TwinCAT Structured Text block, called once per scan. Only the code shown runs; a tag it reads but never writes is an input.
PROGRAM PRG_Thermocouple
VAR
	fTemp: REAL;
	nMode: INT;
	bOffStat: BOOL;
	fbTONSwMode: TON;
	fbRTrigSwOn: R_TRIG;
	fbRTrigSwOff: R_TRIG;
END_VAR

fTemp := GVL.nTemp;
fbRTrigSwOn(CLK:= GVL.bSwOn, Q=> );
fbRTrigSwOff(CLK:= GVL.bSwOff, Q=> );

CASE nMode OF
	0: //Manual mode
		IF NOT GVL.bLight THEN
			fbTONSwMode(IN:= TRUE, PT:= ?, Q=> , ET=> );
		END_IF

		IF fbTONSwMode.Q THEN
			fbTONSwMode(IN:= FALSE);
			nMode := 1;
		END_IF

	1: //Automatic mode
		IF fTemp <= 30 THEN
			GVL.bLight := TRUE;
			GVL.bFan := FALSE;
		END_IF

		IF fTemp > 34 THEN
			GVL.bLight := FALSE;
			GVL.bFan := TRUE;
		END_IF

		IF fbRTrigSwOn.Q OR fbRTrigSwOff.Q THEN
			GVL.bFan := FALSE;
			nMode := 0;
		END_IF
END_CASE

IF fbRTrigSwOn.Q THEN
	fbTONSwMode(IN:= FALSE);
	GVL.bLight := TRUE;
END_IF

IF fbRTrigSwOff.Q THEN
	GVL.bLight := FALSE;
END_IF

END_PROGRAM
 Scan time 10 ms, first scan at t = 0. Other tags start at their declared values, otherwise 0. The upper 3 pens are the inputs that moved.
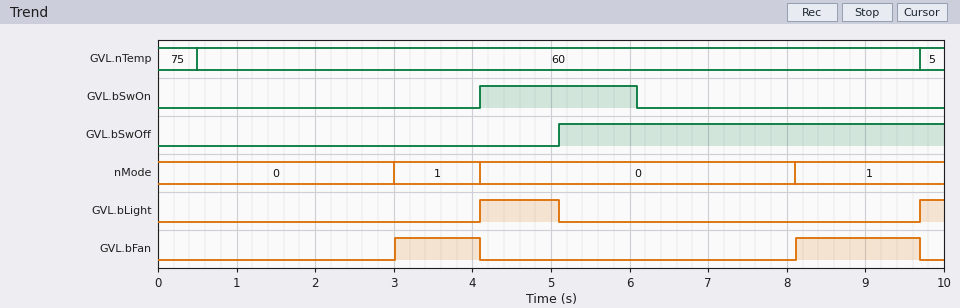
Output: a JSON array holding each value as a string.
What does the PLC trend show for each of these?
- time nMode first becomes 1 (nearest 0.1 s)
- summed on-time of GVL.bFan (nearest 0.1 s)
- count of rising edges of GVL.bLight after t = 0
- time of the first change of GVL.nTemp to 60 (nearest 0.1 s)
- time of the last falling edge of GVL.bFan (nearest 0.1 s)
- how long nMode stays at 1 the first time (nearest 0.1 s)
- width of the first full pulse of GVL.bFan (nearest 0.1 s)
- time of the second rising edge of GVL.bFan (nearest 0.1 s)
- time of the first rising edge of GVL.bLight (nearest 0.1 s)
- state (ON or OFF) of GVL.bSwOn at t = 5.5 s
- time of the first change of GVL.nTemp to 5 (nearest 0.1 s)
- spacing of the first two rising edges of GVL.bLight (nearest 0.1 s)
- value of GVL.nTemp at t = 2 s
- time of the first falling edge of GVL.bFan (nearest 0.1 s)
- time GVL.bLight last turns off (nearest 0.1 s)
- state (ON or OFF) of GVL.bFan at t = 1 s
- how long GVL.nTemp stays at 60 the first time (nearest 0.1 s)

["3.0 s", "2.7 s", "2", "0.5 s", "9.7 s", "1.1 s", "1.1 s", "8.1 s", "4.1 s", "ON", "9.7 s", "5.6 s", "60", "4.1 s", "5.1 s", "OFF", "9.2 s"]
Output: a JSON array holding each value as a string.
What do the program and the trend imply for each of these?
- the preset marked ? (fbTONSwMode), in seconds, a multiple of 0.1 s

["3.0 s"]
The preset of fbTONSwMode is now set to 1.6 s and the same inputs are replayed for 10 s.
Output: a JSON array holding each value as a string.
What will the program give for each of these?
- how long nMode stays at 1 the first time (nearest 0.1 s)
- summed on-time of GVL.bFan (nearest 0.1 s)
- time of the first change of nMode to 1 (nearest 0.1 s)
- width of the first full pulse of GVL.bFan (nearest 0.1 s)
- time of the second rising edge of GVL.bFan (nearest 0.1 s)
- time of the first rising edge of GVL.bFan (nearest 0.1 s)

["2.5 s", "5.5 s", "1.6 s", "2.5 s", "6.7 s", "1.6 s"]
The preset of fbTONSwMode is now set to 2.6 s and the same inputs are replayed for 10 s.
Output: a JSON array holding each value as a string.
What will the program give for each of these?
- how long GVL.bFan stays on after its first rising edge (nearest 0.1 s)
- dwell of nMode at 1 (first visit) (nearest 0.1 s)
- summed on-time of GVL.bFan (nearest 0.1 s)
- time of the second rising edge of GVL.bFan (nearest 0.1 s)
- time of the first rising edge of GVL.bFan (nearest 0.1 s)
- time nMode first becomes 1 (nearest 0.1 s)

["1.5 s", "1.5 s", "3.5 s", "7.7 s", "2.6 s", "2.6 s"]
